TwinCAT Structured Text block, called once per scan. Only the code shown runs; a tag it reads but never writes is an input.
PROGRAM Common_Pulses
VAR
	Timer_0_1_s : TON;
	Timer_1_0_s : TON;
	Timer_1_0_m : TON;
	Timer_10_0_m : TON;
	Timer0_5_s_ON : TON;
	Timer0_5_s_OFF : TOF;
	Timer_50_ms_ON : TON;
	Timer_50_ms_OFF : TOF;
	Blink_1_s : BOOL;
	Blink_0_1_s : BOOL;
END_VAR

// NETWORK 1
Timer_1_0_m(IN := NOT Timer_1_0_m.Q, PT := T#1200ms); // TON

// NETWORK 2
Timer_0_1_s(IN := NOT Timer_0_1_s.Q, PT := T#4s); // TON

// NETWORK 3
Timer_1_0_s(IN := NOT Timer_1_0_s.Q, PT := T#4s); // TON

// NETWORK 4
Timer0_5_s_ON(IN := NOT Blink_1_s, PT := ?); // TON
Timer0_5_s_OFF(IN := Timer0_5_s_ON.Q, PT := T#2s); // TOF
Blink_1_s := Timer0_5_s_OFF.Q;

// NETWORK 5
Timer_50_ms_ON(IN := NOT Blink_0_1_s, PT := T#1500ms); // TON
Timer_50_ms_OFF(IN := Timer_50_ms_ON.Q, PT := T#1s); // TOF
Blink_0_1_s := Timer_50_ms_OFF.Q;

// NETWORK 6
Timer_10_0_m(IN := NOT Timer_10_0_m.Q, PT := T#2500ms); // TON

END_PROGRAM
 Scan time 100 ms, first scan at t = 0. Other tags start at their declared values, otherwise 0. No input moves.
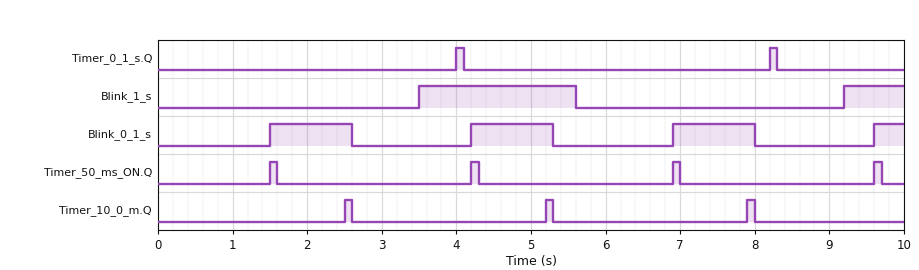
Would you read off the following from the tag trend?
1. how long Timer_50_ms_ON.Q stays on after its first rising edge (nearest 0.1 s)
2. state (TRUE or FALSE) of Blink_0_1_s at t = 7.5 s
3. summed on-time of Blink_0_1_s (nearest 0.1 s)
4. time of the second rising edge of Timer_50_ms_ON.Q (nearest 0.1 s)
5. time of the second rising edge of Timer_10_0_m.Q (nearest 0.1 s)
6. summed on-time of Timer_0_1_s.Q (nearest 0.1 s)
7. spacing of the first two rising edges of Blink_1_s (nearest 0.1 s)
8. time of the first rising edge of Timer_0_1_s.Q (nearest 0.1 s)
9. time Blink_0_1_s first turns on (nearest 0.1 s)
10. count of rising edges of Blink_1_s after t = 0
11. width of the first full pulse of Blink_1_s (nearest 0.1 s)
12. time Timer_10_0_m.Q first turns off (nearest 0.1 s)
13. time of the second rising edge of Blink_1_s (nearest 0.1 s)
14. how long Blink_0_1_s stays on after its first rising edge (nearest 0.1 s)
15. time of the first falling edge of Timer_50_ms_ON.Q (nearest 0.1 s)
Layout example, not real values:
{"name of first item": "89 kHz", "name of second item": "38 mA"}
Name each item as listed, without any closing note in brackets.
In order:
{"how long Timer_50_ms_ON.Q stays on after its first rising edge": "0.1 s", "state (TRUE or FALSE) of Blink_0_1_s at t = 7.5 s": "TRUE", "summed on-time of Blink_0_1_s": "3.7 s", "time of the second rising edge of Timer_50_ms_ON.Q": "4.2 s", "time of the second rising edge of Timer_10_0_m.Q": "5.2 s", "summed on-time of Timer_0_1_s.Q": "0.2 s", "spacing of the first two rising edges of Blink_1_s": "5.7 s", "time of the first rising edge of Timer_0_1_s.Q": "4.0 s", "time Blink_0_1_s first turns on": "1.5 s", "count of rising edges of Blink_1_s after t = 0": "2", "width of the first full pulse of Blink_1_s": "2.1 s", "time Timer_10_0_m.Q first turns off": "2.6 s", "time of the second rising edge of Blink_1_s": "9.2 s", "how long Blink_0_1_s stays on after its first rising edge": "1.1 s", "time of the first falling edge of Timer_50_ms_ON.Q": "1.6 s"}
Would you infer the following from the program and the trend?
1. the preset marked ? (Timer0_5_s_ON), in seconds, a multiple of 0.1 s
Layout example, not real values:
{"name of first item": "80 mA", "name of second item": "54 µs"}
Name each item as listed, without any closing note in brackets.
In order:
{"the preset marked ? (Timer0_5_s_ON), in seconds, a multiple of 0.1 s": "3.5 s"}
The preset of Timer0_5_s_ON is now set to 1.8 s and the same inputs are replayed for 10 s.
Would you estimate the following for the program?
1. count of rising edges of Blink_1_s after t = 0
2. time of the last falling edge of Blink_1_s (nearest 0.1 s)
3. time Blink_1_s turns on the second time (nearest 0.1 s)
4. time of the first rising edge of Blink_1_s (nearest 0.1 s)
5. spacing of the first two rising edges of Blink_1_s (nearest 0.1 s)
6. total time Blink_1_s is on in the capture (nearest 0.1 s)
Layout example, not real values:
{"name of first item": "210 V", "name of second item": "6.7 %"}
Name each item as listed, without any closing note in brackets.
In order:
{"count of rising edges of Blink_1_s after t = 0": "3", "time of the last falling edge of Blink_1_s": "7.9 s", "time Blink_1_s turns on the second time": "5.8 s", "time of the first rising edge of Blink_1_s": "1.8 s", "spacing of the first two rising edges of Blink_1_s": "4.0 s", "total time Blink_1_s is on in the capture": "4.4 s"}
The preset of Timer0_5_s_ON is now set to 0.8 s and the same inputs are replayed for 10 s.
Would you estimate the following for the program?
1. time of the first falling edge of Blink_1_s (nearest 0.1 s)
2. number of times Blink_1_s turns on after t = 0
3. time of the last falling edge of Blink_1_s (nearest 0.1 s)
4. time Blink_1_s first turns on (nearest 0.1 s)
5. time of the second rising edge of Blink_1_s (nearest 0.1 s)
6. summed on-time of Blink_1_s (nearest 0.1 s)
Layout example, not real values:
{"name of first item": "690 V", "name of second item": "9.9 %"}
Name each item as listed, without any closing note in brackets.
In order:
{"time of the first falling edge of Blink_1_s": "2.9 s", "number of times Blink_1_s turns on after t = 0": "4", "time of the last falling edge of Blink_1_s": "8.9 s", "time Blink_1_s first turns on": "0.8 s", "time of the second rising edge of Blink_1_s": "3.8 s", "summed on-time of Blink_1_s": "6.5 s"}
